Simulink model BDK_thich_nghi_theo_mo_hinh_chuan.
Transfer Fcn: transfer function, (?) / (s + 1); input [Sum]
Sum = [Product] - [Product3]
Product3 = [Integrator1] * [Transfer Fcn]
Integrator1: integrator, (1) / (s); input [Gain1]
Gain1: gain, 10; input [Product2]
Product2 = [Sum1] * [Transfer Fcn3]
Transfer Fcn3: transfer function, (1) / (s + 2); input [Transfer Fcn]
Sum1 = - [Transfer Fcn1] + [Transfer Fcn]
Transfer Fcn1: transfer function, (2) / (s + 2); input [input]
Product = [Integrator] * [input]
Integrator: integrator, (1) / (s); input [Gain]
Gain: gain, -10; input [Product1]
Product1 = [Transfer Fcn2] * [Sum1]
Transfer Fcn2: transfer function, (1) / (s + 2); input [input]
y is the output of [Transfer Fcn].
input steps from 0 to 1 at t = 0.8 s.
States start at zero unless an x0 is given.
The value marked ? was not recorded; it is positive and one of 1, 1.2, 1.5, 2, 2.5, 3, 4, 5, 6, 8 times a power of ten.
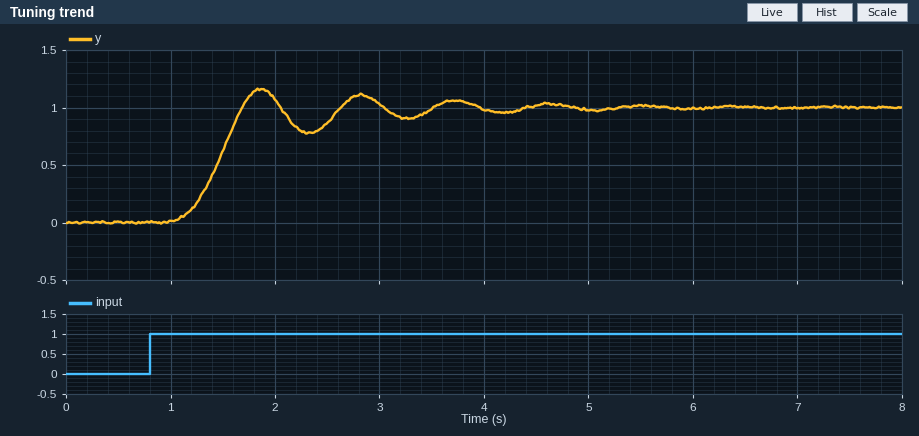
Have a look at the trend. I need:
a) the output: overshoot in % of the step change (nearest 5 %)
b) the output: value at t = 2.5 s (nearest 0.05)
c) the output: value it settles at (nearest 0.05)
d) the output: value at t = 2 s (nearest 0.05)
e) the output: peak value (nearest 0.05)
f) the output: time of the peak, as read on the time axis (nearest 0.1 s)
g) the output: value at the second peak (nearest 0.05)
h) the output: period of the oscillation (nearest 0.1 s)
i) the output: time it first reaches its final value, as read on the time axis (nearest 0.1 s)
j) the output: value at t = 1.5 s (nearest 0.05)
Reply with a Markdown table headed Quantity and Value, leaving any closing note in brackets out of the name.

| Quantity | Value |
|---|---|
| the output: overshoot in % of the step change | 15 % |
| the output: value at t = 2.5 s | 0.85 |
| the output: value it settles at | 1.00 |
| the output: value at t = 2 s | 1.05 |
| the output: peak value | 1.15 |
| the output: time of the peak, as read on the time axis | 1.9 s |
| the output: value at the second peak | 1.10 |
| the output: period of the oscillation | 1.0 s |
| the output: time it first reaches its final value, as read on the time axis | 1.7 s |
| the output: value at t = 1.5 s | 0.60 |
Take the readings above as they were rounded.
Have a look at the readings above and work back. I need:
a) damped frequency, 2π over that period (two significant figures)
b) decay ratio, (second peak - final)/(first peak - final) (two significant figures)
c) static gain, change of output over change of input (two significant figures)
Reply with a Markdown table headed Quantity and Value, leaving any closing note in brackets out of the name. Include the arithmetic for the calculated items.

| Quantity | Value |
|---|---|
| damped frequency, 2π over that period | 2π / 1 = 6.3 rad/s |
| decay ratio, (second peak - final)/(first peak - final) | (1.1 - 1) / (1.15 - 1) = 0.67 |
| static gain, change of output over change of input | (1 - 0) / (1 - 0) = 1.0 |
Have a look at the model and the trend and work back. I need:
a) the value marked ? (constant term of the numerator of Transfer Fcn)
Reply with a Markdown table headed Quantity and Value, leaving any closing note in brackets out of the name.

| Quantity | Value |
|---|---|
| the value marked ? | 5 |
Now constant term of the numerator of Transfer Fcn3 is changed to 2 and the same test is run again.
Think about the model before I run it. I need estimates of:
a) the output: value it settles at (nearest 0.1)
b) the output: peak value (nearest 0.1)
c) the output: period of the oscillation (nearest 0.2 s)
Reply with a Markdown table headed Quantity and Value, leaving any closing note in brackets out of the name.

| Quantity | Value |
|---|---|
| the output: value it settles at | 1.0 |
| the output: peak value | 1.1 |
| the output: period of the oscillation | 0.8 s |
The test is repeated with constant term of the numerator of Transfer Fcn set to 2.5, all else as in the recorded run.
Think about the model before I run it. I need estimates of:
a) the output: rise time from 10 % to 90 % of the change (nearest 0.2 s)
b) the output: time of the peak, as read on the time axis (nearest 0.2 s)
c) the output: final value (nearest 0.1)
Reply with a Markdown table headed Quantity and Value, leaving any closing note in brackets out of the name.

| Quantity | Value |
|---|---|
| the output: rise time from 10 % to 90 % of the change | 0.6 s |
| the output: time of the peak, as read on the time axis | 2.2 s |
| the output: final value | 1.0 |
